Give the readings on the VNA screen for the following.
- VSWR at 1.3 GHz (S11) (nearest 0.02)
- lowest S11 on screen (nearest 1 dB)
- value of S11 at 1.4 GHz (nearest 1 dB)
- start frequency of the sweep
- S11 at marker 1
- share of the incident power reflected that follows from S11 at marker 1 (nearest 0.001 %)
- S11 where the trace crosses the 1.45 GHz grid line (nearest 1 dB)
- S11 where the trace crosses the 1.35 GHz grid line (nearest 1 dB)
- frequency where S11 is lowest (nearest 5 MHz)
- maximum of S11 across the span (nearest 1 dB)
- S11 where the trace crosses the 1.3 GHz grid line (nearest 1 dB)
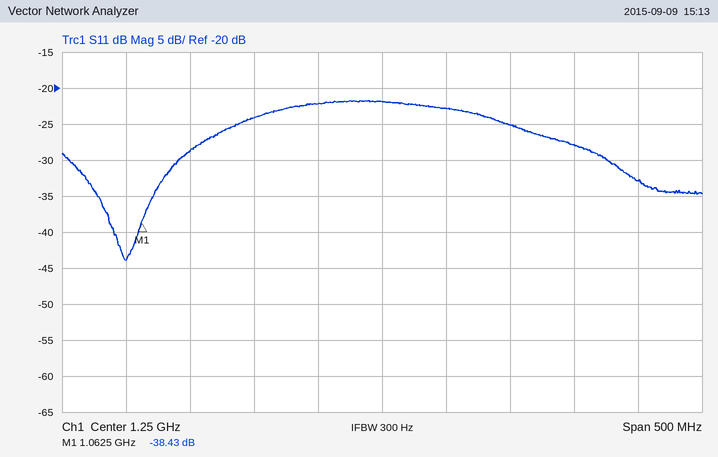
1.16
-44 dB
-28 dB
1 GHz
-38.43 dB
0.014 %
-33 dB
-25 dB
1.050 GHz
-22 dB
-23 dB
